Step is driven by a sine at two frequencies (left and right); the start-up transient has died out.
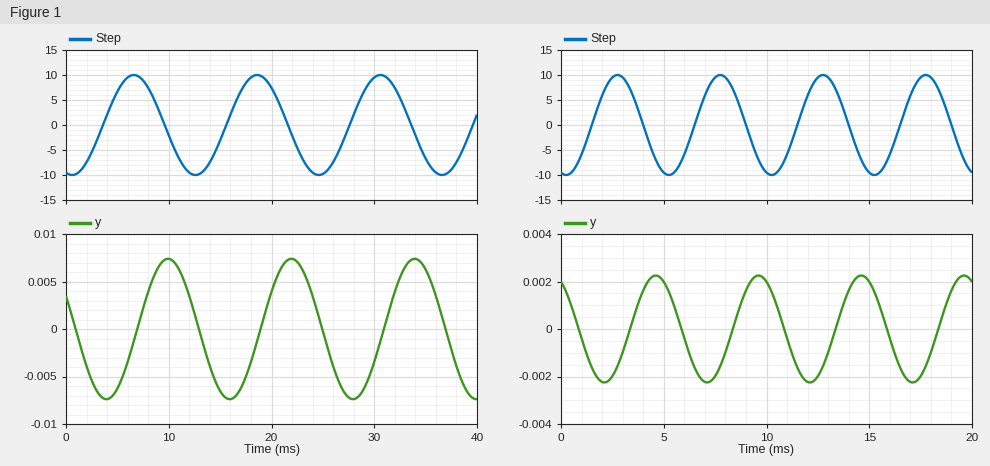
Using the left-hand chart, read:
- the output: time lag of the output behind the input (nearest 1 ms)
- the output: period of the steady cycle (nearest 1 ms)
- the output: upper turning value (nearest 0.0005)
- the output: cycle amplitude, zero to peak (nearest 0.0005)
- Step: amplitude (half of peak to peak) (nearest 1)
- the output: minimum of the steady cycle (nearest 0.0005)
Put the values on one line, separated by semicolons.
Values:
3 ms; 12 ms; 0.0075; 0.0075; 10; -0.0075
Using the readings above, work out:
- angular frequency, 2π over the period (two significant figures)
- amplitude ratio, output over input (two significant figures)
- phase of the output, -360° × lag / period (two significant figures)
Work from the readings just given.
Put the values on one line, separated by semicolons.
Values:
0.52 rad/ms; 0.00075; -90°
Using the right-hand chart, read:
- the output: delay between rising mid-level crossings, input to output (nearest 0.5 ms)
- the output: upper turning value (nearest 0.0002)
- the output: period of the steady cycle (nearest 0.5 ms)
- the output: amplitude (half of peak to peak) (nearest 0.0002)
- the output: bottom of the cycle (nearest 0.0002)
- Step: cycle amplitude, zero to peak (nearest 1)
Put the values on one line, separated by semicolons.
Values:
2.0 ms; 0.0022; 5.0 ms; 0.0022; -0.0022; 10
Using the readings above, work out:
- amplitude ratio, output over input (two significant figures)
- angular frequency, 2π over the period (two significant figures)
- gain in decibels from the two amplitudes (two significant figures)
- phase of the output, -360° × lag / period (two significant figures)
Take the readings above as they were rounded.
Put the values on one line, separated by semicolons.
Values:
0.00022; 1.3 rad/ms; -73 dB; -140°
